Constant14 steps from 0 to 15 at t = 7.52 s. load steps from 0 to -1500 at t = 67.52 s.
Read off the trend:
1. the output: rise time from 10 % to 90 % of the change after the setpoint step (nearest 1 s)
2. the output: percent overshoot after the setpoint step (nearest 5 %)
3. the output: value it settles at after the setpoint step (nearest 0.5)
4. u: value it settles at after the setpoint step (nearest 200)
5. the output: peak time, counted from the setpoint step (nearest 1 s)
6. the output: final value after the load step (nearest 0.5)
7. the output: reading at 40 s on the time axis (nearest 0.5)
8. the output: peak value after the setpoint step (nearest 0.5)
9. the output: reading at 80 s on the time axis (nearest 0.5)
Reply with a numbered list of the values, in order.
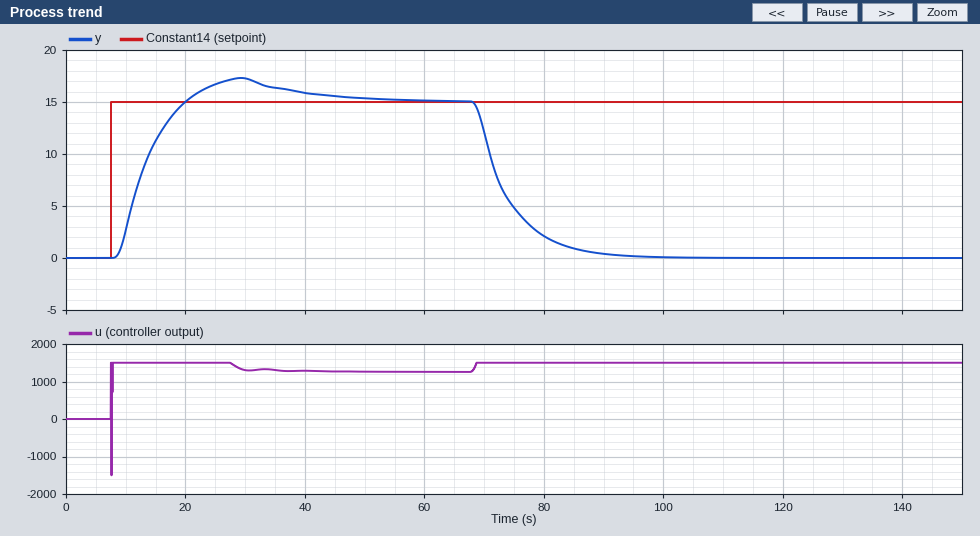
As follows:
1. 8 s
2. 15 %
3. 15.0
4. 1200
5. 22 s
6. 0.0
7. 16.0
8. 17.5
9. 2.0
